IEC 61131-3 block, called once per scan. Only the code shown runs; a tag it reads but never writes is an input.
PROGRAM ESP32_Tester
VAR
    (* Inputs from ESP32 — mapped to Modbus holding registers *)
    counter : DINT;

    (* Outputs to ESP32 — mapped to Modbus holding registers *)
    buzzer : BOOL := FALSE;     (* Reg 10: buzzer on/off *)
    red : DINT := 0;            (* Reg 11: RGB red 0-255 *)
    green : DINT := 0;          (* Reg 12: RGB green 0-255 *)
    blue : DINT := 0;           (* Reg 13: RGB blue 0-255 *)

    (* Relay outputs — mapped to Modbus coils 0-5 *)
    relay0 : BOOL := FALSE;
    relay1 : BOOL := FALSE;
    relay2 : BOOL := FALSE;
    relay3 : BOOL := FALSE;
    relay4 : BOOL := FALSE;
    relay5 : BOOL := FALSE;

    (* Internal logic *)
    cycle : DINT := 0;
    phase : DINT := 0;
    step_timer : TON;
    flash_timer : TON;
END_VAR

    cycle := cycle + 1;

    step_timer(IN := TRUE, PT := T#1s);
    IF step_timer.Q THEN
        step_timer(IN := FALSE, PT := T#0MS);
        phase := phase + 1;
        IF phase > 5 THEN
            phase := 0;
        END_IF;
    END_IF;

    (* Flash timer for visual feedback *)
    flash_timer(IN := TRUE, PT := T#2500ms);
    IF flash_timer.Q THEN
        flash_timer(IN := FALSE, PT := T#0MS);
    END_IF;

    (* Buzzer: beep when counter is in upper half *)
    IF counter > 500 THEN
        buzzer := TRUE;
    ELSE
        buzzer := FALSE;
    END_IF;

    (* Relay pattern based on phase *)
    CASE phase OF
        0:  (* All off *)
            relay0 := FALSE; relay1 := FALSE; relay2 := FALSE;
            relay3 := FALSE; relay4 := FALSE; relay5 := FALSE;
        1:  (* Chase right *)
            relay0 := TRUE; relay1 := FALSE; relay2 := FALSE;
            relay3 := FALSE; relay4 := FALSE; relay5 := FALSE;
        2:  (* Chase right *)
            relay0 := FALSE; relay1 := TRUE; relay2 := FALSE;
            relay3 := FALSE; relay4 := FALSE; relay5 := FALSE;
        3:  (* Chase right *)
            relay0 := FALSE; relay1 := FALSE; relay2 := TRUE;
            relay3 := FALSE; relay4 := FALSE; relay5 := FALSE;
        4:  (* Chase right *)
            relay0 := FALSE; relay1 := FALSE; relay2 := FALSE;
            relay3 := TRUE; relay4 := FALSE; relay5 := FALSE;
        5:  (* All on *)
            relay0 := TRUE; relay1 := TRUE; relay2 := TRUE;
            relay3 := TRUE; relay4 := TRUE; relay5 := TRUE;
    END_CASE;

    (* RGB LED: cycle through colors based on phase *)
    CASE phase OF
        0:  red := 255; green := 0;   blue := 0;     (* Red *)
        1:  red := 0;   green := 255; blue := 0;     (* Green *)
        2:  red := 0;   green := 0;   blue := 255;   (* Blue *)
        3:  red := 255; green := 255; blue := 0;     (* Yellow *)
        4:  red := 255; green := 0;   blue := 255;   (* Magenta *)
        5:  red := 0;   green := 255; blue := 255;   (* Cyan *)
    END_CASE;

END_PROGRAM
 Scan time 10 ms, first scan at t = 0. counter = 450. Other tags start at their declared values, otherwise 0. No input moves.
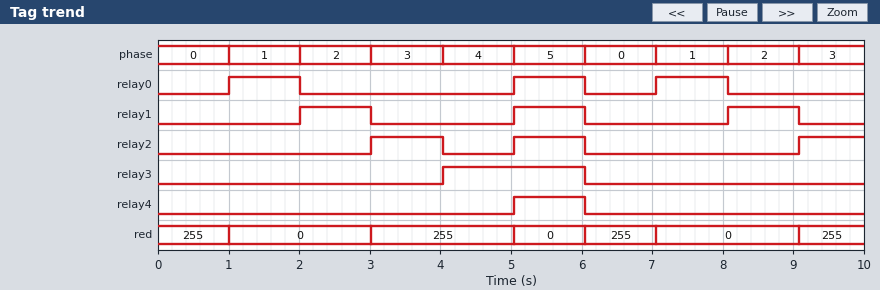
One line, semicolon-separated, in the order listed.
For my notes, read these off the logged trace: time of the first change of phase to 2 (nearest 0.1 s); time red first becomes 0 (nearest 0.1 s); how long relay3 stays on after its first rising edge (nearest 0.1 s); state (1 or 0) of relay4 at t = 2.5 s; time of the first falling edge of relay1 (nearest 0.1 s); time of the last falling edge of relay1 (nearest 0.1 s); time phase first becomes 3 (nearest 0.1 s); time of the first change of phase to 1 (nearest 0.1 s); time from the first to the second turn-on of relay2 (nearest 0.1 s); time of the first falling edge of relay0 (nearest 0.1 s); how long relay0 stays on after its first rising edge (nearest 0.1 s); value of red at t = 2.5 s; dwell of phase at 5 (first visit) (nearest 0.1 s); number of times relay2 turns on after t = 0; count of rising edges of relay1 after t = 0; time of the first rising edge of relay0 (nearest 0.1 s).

2.0 s; 1.0 s; 2.0 s; 0; 3.0 s; 9.1 s; 3.0 s; 1.0 s; 2.0 s; 2.0 s; 1.0 s; 0; 1.0 s; 3; 3; 1.0 s
